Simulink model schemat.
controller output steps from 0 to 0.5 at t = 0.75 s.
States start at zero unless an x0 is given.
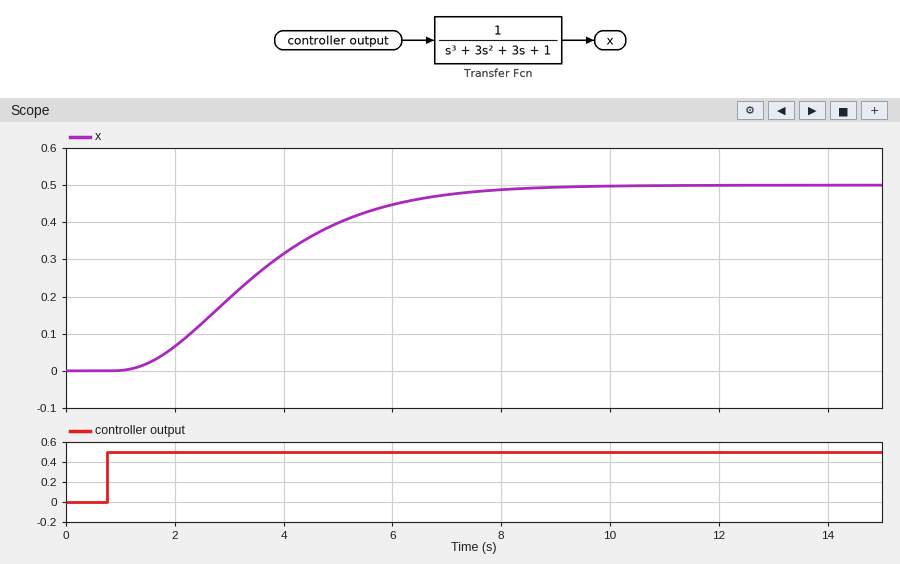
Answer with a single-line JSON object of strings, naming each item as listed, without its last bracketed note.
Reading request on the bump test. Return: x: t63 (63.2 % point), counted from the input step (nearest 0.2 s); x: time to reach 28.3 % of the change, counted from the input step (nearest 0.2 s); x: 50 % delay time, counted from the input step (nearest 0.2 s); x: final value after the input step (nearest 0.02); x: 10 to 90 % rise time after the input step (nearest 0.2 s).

{"x: t63 (63.2 % point), counted from the input step": "3.2 s", "x: time to reach 28.3 % of the change, counted from the input step": "1.8 s", "x: 50 % delay time, counted from the input step": "2.6 s", "x: final value after the input step": "0.50", "x: 10 to 90 % rise time after the input step": "4.2 s"}
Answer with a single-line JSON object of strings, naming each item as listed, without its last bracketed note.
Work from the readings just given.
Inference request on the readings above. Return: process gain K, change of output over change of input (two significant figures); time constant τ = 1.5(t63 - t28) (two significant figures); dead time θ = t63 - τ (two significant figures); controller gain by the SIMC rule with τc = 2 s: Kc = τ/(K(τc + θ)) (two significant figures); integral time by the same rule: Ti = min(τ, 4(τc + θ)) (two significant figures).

{"process gain K, change of output over change of input": "1.0", "time constant τ = 1.5(t63 - t28)": "2.1 s", "dead time θ = t63 - τ": "1.1 s", "controller gain by the SIMC rule with τc = 2 s: Kc = τ/(K(τc + θ))": "0.68", "integral time by the same rule: Ti = min(τ, 4(τc + θ))": "2.1 s"}
